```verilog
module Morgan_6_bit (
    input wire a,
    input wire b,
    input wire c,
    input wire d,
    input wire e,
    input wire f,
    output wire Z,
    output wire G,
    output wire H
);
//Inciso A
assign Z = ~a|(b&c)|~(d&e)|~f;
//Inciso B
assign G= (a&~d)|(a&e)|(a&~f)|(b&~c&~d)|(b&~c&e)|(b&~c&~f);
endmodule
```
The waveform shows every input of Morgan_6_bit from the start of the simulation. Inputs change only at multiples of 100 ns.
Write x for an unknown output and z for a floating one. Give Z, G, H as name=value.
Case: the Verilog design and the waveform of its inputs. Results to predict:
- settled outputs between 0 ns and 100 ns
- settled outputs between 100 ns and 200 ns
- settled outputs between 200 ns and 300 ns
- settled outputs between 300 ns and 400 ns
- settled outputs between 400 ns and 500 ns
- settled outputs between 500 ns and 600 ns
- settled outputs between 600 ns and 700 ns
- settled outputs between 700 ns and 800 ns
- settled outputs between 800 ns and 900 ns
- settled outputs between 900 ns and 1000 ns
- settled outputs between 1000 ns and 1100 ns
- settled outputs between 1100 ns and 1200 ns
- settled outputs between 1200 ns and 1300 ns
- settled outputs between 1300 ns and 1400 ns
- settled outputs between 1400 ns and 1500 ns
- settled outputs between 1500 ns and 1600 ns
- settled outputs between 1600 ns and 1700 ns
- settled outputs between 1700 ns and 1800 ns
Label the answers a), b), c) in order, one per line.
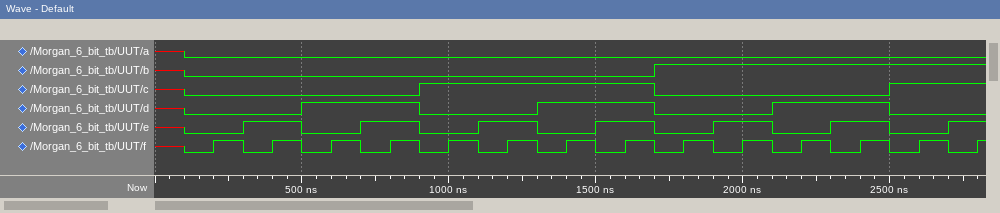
a) Z=x, G=x, H=z
b) Z=1, G=0, H=z
c) Z=1, G=0, H=z
d) Z=1, G=0, H=z
e) Z=1, G=0, H=z
f) Z=1, G=0, H=z
g) Z=1, G=0, H=z
h) Z=1, G=0, H=z
i) Z=1, G=0, H=z
j) Z=1, G=0, H=z
k) Z=1, G=0, H=z
l) Z=1, G=0, H=z
m) Z=1, G=0, H=z
n) Z=1, G=0, H=z
o) Z=1, G=0, H=z
p) Z=1, G=0, H=z
q) Z=1, G=0, H=z
r) Z=1, G=1, H=z
